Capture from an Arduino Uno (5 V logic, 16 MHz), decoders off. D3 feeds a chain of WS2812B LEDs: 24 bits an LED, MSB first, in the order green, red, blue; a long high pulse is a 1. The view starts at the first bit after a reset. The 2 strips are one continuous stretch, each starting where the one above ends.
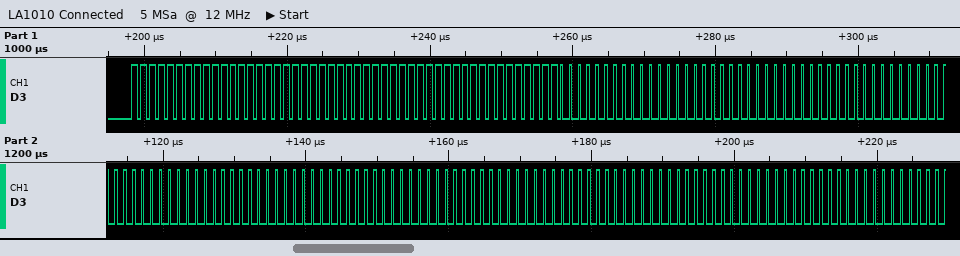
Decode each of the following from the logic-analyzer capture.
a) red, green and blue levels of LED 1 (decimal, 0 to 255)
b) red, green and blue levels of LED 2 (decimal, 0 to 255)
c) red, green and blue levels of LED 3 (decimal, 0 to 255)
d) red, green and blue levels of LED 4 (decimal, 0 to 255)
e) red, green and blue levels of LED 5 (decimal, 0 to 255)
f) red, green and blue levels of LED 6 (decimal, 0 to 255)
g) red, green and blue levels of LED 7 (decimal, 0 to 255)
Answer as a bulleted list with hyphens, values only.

- 255, 255, 255
- 255, 255, 255
- 0, 0, 0
- 0, 0, 0
- 0, 0, 0
- 0, 0, 0
- 0, 0, 0
